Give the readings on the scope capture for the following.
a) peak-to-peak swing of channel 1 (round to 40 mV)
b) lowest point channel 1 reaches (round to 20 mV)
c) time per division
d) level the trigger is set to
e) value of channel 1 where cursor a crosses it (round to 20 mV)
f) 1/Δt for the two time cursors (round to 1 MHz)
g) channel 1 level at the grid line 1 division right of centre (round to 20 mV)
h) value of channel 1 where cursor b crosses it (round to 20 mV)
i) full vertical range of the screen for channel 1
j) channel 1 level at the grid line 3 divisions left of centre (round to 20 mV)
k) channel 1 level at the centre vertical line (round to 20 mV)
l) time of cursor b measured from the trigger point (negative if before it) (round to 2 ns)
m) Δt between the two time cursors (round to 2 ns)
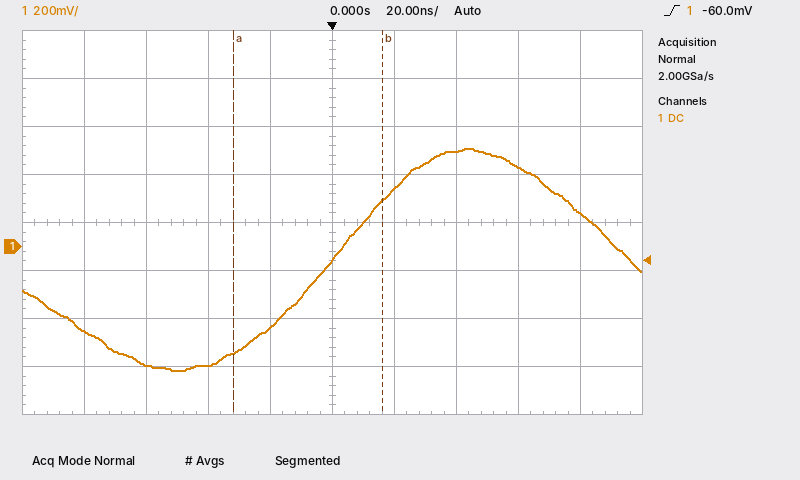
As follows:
920 mV
-520 mV
20 ns
-60.0 mV
-440 mV
21 MHz
240 mV
200 mV
1.6 V
-500 mV
-60 mV
+16 ns
48 ns
